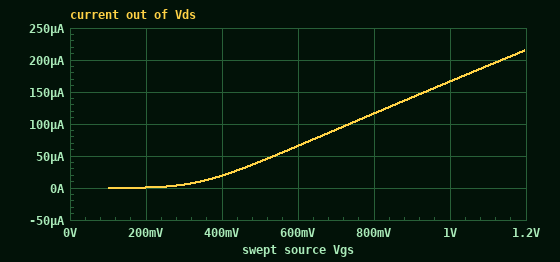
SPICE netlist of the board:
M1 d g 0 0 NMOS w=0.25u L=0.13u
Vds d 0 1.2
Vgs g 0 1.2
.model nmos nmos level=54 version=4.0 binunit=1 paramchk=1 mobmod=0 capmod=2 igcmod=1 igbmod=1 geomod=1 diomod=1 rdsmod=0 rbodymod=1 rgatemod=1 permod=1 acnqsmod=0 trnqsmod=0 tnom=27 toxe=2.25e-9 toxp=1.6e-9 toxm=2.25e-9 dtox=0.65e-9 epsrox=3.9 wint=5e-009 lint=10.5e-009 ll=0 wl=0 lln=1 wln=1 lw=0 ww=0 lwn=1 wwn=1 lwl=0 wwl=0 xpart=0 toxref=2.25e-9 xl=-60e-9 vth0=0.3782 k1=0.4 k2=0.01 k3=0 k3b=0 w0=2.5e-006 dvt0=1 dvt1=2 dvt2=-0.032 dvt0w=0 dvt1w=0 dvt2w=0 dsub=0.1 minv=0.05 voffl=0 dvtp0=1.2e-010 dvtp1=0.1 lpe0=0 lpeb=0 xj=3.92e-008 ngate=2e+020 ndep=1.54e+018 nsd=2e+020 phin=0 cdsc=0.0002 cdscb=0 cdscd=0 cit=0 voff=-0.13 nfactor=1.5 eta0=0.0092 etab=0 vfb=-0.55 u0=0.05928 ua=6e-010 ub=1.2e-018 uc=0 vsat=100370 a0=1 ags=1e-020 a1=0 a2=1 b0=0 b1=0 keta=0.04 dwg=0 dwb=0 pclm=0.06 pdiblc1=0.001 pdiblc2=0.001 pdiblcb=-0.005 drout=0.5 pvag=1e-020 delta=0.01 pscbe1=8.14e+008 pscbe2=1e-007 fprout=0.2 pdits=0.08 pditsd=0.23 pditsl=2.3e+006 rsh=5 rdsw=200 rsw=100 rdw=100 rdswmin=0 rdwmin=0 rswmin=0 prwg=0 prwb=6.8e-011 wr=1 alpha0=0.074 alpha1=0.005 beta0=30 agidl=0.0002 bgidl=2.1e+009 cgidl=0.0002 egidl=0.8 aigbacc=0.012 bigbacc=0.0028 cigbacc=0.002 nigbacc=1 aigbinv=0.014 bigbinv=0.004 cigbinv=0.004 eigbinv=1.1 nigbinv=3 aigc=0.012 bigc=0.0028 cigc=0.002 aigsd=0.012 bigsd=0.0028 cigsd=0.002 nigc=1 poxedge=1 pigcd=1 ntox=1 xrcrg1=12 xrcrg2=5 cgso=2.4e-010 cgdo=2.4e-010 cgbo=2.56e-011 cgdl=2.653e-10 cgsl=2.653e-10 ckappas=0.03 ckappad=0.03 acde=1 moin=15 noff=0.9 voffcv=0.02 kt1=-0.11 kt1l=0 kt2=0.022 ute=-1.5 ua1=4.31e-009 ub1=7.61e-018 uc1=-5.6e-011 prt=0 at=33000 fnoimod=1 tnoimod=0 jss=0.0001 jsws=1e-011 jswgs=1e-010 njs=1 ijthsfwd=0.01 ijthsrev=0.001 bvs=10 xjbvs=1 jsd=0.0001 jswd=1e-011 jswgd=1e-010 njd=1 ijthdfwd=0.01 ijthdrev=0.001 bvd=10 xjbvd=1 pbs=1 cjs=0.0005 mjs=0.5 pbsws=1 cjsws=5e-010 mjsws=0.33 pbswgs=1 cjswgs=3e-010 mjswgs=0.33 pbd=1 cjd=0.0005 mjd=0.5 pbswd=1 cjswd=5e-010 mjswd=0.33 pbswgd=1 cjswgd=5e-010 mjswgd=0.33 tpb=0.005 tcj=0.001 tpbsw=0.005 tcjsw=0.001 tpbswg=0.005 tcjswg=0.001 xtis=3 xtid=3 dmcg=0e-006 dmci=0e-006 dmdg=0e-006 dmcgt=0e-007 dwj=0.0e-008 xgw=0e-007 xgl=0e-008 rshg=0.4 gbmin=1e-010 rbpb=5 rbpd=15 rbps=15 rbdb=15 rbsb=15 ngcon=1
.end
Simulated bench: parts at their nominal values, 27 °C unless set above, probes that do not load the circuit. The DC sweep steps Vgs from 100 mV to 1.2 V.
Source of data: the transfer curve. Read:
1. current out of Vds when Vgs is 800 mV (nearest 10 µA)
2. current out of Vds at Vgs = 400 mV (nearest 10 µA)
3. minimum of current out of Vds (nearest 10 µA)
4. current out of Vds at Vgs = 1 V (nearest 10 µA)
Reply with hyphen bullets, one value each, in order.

- 120 µA
- 20 µA
- 0 A
- 170 µA
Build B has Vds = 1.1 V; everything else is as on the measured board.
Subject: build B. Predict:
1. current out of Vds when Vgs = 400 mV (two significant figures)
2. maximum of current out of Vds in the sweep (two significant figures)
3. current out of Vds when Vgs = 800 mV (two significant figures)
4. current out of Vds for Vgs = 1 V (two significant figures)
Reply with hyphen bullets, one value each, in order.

- 18 µA
- 210 µA
- 110 µA
- 160 µA
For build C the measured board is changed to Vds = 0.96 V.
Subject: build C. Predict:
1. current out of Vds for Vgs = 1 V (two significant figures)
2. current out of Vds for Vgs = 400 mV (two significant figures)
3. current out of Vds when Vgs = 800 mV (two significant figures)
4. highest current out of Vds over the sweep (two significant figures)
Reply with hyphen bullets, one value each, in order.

- 160 µA
- 16 µA
- 110 µA
- 210 µA
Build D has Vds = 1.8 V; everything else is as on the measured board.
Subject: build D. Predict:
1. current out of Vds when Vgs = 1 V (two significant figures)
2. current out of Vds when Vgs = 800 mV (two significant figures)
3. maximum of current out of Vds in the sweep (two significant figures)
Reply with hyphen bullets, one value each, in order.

- 180 µA
- 130 µA
- 230 µA
